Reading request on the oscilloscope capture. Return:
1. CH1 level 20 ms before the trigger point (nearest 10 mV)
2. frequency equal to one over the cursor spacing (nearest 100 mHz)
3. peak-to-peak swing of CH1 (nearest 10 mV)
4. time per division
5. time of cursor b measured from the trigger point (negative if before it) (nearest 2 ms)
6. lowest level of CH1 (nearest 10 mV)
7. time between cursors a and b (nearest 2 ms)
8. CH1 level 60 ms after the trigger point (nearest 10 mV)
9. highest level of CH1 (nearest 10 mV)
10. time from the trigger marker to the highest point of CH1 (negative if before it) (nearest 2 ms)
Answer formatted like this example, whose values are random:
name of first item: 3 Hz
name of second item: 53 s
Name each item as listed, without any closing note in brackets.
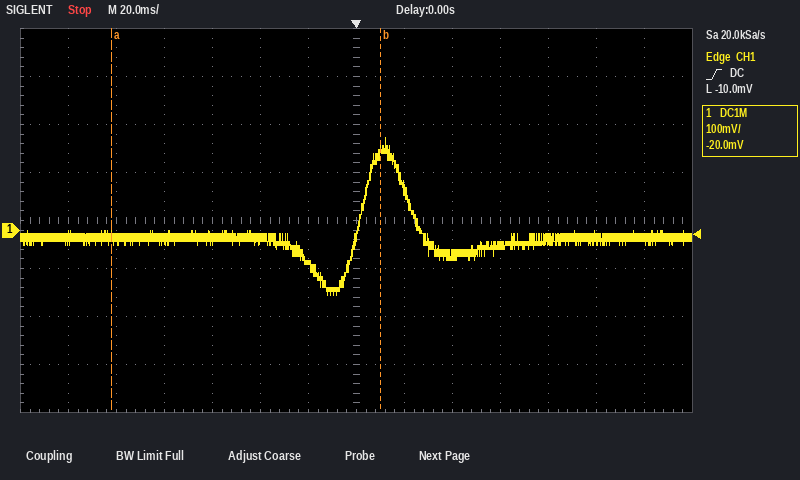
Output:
CH1 level 20 ms before the trigger point: -70 mV
frequency equal to one over the cursor spacing: 8.9 Hz
peak-to-peak swing of CH1: 330 mV
time per division: 20 ms
time of cursor b measured from the trigger point (negative if before it): +10 ms
lowest level of CH1: -140 mV
time between cursors a and b: 112 ms
CH1 level 60 ms after the trigger point: -30 mV
highest level of CH1: 190 mV
time from the trigger marker to the highest point of CH1 (negative if before it): +12 ms
